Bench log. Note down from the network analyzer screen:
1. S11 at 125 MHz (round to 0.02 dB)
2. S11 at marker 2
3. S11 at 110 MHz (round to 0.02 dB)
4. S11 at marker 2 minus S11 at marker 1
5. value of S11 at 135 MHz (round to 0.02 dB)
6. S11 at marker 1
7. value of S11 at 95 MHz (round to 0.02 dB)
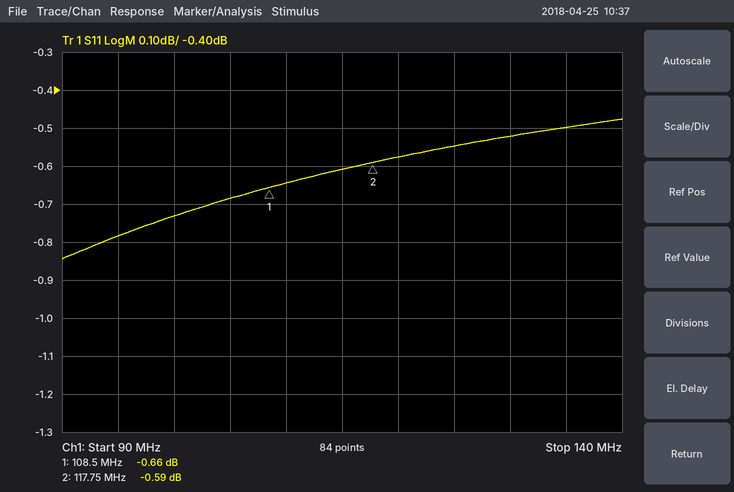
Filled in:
-0.54 dB
-0.59 dB
-0.64 dB
0.07 dB
-0.50 dB
-0.66 dB
-0.78 dB
